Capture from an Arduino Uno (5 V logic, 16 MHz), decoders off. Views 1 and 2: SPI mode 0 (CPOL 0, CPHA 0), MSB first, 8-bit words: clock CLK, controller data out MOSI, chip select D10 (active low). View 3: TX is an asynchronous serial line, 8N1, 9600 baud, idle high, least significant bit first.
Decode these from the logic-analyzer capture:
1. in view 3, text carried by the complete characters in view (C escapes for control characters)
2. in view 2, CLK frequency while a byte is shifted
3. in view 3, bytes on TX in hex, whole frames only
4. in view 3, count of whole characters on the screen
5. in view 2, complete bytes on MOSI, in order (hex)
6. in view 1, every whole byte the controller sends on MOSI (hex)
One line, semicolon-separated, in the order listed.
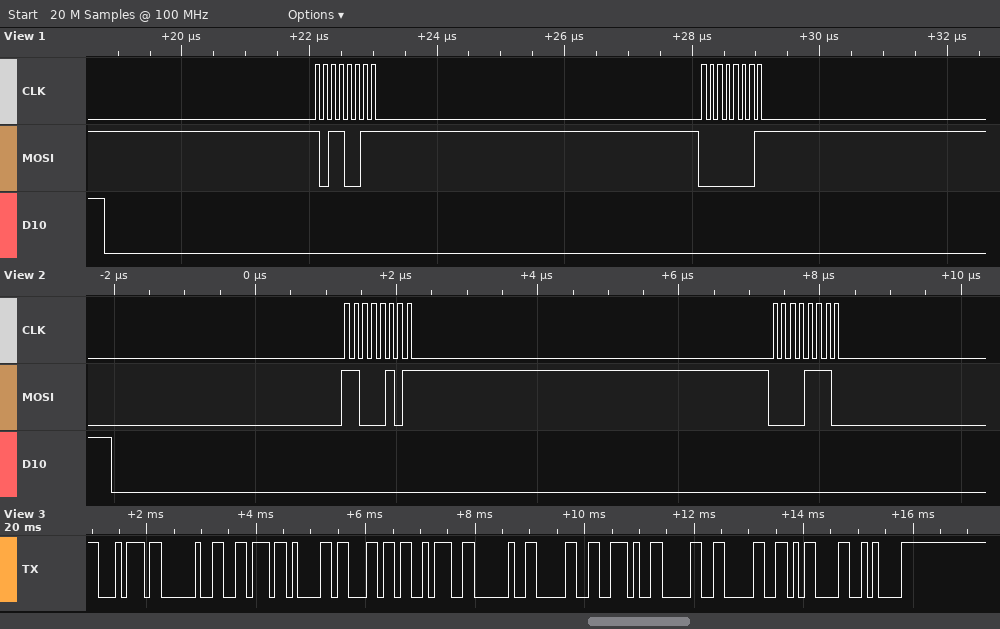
"t val: 0.00\r\n"; 8 MHz; 74 20 76 61 6C 3A 20 30 2E 30 30 0D 0A; 13; C5 0E; B3 01
